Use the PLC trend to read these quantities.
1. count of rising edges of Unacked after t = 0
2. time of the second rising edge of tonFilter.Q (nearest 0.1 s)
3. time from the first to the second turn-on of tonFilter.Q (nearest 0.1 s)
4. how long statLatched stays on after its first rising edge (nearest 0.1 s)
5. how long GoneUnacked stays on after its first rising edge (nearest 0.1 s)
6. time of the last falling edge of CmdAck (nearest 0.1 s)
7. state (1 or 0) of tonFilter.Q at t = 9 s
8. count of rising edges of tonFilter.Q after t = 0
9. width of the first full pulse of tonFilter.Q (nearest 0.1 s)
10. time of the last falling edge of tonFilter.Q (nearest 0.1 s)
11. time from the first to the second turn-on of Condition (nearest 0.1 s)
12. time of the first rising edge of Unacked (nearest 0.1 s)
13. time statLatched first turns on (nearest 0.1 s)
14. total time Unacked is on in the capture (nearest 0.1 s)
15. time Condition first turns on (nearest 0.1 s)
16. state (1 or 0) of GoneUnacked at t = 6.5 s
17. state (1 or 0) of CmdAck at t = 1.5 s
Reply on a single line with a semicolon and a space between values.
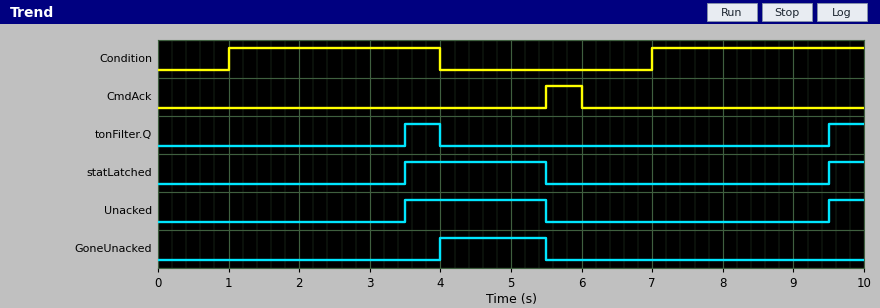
2; 9.5 s; 6.0 s; 2.0 s; 1.5 s; 6.0 s; 0; 2; 0.5 s; 4.0 s; 6.0 s; 3.5 s; 3.5 s; 2.5 s; 1.0 s; 0; 0
